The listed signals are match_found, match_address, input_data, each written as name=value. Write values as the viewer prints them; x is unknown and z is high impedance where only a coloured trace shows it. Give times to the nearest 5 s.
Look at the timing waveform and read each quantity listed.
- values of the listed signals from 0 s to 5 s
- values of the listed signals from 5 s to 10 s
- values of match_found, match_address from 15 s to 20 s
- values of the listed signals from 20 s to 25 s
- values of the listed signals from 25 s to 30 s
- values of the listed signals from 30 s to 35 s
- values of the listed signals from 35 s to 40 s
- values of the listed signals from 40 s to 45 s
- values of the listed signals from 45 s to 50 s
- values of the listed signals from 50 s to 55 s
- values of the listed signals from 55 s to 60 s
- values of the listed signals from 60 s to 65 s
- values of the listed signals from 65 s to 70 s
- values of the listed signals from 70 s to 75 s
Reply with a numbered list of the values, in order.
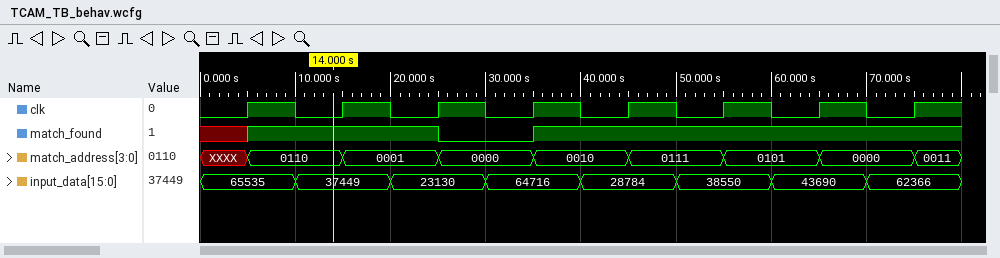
1. match_found=x, match_address=XXXX, input_data=65535
2. match_found=1, match_address=0110, input_data=65535
3. match_found=1, match_address=0001
4. match_found=1, match_address=0001, input_data=23130
5. match_found=0, match_address=0000, input_data=23130
6. match_found=0, match_address=0000, input_data=64716
7. match_found=1, match_address=0010, input_data=64716
8. match_found=1, match_address=0010, input_data=28784
9. match_found=1, match_address=0111, input_data=28784
10. match_found=1, match_address=0111, input_data=38550
11. match_found=1, match_address=0101, input_data=38550
12. match_found=1, match_address=0101, input_data=43690
13. match_found=1, match_address=0000, input_data=43690
14. match_found=1, match_address=0000, input_data=62366
